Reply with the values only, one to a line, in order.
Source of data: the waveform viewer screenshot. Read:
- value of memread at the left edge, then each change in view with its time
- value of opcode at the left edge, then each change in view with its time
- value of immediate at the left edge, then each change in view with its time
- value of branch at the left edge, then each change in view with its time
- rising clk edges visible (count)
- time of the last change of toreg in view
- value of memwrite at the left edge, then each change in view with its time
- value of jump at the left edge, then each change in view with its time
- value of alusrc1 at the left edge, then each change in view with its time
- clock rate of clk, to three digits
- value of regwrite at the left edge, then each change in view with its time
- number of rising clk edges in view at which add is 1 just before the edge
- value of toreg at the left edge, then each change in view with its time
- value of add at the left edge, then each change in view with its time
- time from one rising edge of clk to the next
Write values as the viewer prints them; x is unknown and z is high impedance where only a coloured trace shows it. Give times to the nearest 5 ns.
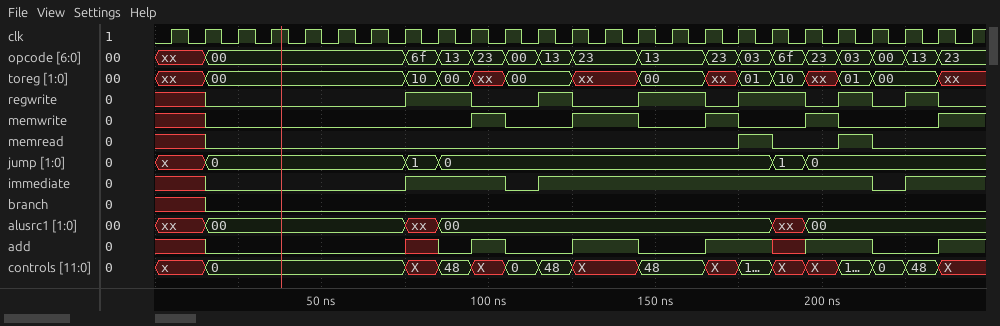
x, 0 at 15 ns, 1 at 175 ns, 0 at 185 ns, 1 at 205 ns, 0 at 215 ns
xx, 00 at 15 ns, 6f at 75 ns, 13 at 85 ns, 23 at 95 ns, 00 at 105 ns, 13 at 115 ns, 23 at 125 ns, 13 at 145 ns, 23 at 165 ns, 03 at 175 ns, 6f at 185 ns, 23 at 195 ns, 03 at 205 ns, 00 at 215 ns, 13 at 225 ns, 23 at 235 ns
x, 0 at 15 ns, 1 at 75 ns, 0 at 105 ns, 1 at 115 ns, 0 at 215 ns, 1 at 225 ns
x, 0 at 15 ns
25
235 ns
x, 0 at 15 ns, 1 at 95 ns, 0 at 105 ns, 1 at 125 ns, 0 at 145 ns, 1 at 165 ns, 0 at 175 ns, 1 at 195 ns, 0 at 205 ns, 1 at 235 ns
x, 0 at 15 ns, 1 at 75 ns, 0 at 85 ns, 1 at 185 ns, 0 at 195 ns
xx, 00 at 15 ns, xx at 75 ns, 00 at 85 ns, xx at 185 ns, 00 at 195 ns
100 MHz
x, 0 at 15 ns, 1 at 75 ns, 0 at 95 ns, 1 at 115 ns, 0 at 125 ns, 1 at 145 ns, 0 at 165 ns, 1 at 175 ns, 0 at 195 ns, 1 at 205 ns, 0 at 215 ns, 1 at 225 ns, 0 at 235 ns
8
xx, 00 at 15 ns, 10 at 75 ns, 00 at 85 ns, xx at 95 ns, 00 at 105 ns, xx at 125 ns, 00 at 145 ns, xx at 165 ns, 01 at 175 ns, 10 at 185 ns, xx at 195 ns, 01 at 205 ns, 00 at 215 ns, xx at 235 ns
x, 0 at 15 ns, x at 75 ns, 0 at 85 ns, 1 at 95 ns, 0 at 105 ns, 1 at 125 ns, 0 at 145 ns, 1 at 165 ns, x at 185 ns, 1 at 195 ns, 0 at 215 ns, 1 at 235 ns
10 ns
